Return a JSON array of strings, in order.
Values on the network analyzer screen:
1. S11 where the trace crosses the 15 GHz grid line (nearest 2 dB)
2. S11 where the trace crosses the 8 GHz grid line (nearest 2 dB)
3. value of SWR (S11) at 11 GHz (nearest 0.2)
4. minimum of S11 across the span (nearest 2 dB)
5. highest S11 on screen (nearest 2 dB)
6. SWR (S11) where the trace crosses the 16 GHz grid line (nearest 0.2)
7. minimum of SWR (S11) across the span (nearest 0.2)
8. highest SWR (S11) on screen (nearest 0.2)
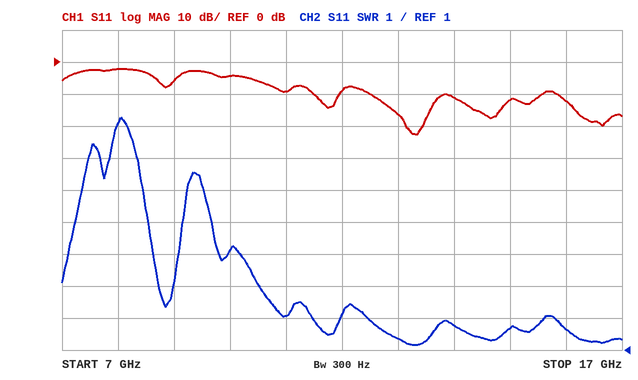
["-12 dB", "-2 dB", "2.0", "-22 dB", "-2 dB", "1.6", "1.2", "8.2"]
